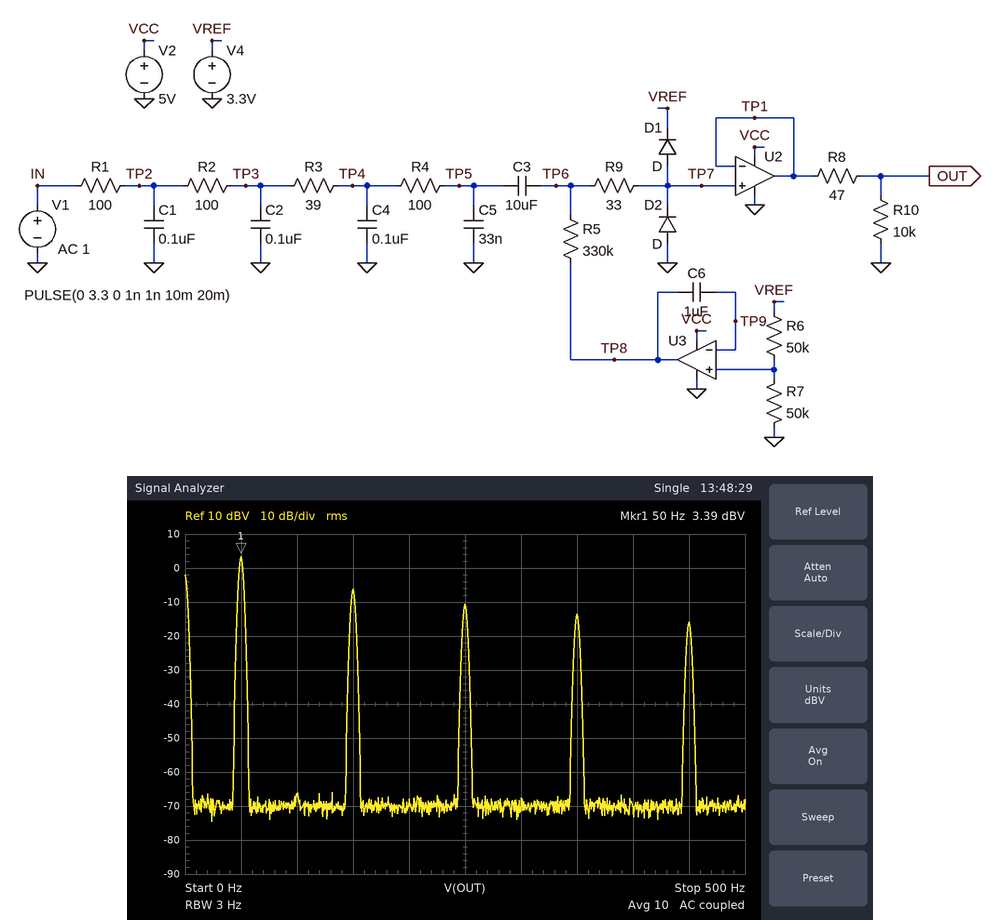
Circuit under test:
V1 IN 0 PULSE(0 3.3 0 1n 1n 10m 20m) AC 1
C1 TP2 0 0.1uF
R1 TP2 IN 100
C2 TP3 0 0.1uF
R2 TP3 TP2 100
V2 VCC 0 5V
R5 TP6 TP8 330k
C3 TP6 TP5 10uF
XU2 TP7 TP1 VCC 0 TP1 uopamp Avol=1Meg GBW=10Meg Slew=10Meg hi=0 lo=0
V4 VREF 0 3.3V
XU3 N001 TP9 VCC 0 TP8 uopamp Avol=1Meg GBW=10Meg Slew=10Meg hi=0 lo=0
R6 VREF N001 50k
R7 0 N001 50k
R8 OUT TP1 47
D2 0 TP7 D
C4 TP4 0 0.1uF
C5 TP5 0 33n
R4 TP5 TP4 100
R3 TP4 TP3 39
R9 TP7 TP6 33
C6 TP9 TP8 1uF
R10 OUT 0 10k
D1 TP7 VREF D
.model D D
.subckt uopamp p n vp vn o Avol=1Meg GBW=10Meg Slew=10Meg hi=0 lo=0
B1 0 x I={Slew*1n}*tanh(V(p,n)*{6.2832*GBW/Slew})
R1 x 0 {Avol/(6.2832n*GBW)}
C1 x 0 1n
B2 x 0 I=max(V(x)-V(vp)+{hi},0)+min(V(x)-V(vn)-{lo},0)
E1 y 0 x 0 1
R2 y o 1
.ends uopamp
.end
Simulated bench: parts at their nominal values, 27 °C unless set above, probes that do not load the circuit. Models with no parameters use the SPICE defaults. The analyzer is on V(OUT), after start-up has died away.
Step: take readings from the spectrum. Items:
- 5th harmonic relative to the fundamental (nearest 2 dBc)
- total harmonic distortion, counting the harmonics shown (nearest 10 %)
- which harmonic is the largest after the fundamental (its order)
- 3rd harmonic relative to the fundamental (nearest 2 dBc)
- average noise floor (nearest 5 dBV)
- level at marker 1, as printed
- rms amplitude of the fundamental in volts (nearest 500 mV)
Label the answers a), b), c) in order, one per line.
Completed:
a) -14 dBc
b) 40 %
c) 3
d) -10 dBc
e) -70 dBV
f) 3.39 dBV
g) 1.5 V
